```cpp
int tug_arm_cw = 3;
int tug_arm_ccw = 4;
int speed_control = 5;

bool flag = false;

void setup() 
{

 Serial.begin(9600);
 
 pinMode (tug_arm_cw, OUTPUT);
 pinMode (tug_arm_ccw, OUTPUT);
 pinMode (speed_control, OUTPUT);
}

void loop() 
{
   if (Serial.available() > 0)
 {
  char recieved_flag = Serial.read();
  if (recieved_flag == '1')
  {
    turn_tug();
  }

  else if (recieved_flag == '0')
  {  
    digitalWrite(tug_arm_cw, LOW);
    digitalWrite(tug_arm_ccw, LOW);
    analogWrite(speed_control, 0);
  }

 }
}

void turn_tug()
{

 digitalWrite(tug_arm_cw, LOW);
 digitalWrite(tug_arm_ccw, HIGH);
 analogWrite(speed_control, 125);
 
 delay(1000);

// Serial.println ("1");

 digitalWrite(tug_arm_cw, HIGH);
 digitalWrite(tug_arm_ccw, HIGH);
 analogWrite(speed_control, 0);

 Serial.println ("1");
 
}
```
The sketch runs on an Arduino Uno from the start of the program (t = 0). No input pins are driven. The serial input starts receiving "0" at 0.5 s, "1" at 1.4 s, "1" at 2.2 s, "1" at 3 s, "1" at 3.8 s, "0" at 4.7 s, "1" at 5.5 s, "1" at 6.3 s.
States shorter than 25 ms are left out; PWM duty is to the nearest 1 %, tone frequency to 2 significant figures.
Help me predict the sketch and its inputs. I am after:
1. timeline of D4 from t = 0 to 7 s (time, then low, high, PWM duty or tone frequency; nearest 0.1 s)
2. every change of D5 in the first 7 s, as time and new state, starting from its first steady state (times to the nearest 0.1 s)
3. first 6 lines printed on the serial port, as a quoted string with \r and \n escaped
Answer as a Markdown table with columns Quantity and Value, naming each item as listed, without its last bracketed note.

| Quantity | Value |
|---|---|
| timeline of D4 from t = 0 to 7 s | 0 s low; 1.4 s high; 5.4 s low; 5.5 s high |
| every change of D5 in the first 7 s, as time and new state, starting from its first steady state | 0 s low; 1.4 s PWM 49 %; 5.4 s low; 5.5 s PWM 49 % |
| first 6 lines printed on the serial port, as a quoted string with \r and \n escaped | "1\r\n1\r\n1\r\n1\r\n1\r\n1\r\n" |
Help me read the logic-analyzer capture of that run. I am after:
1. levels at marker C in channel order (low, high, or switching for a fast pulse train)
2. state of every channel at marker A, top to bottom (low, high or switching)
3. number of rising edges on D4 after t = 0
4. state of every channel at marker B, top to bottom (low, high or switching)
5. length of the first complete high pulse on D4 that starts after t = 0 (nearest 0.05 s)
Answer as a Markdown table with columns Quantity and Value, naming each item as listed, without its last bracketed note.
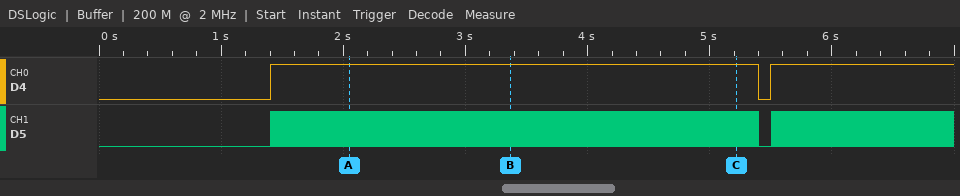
| Quantity | Value |
|---|---|
| levels at marker C in channel order | D4 high, D5 switching |
| state of every channel at marker A, top to bottom | D4 high, D5 switching |
| number of rising edges on D4 after t = 0 | 2 |
| state of every channel at marker B, top to bottom | D4 high, D5 switching |
| length of the first complete high pulse on D4 that starts after t = 0 | 4.00 s |
